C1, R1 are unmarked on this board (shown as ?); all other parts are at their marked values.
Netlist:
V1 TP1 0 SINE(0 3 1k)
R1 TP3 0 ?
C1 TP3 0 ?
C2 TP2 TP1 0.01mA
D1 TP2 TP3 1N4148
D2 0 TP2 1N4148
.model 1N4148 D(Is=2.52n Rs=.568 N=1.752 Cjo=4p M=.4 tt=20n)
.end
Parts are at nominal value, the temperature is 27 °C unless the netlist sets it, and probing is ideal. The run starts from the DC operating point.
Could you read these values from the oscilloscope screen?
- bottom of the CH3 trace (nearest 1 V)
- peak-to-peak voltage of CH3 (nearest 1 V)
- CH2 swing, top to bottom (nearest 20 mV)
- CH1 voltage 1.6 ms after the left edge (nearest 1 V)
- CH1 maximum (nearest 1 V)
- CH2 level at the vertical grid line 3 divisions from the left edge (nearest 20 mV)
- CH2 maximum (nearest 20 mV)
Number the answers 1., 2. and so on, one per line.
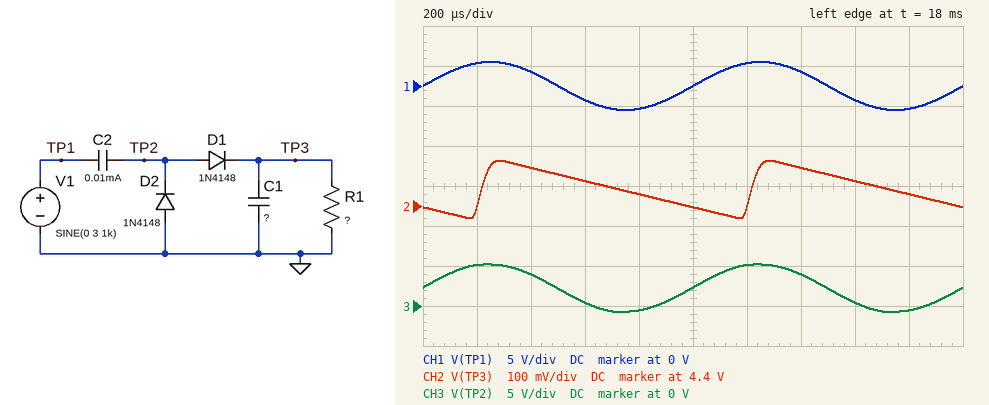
1. -1 V
2. 6 V
3. 140 mV
4. -2 V
5. 3 V
6. 4.46 V
7. 4.52 V
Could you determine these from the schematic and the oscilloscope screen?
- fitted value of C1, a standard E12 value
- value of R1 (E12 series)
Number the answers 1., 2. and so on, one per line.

1. 8.2 µF
2. 3.3 kΩ
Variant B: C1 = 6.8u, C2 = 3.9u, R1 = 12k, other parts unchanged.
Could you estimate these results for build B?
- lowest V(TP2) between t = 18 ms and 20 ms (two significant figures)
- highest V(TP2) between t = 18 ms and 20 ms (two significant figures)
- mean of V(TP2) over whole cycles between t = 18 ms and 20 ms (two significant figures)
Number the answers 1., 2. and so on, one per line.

1. -680 mV
2. 5.3 V
3. 2.3 V
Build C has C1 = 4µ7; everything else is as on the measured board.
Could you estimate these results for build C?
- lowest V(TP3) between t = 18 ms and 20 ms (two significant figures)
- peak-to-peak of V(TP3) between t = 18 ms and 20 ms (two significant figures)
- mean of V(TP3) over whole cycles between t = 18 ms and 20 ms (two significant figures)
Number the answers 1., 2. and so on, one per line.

1. 4.3 V
2. 250 mV
3. 4.4 V
